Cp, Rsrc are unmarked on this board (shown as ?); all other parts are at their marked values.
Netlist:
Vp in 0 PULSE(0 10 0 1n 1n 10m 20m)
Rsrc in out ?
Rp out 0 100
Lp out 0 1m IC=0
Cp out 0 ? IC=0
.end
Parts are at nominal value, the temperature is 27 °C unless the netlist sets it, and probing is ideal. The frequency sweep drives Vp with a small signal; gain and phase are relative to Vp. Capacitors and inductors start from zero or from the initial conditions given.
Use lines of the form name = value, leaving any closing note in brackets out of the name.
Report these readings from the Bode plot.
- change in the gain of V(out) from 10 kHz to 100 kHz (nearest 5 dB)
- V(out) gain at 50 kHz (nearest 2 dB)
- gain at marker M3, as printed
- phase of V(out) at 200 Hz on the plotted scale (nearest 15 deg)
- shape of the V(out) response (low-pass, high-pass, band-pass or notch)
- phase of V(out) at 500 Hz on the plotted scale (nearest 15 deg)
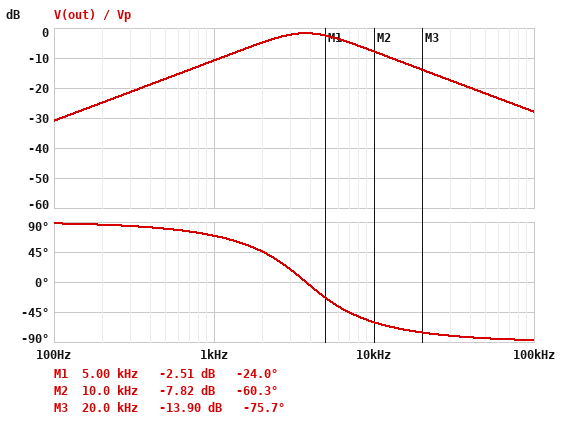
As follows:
change in the gain of V(out) from 10 kHz to 100 kHz = -20 dB
V(out) gain at 50 kHz = -22 dB
gain at marker M3, as printed = -13.90 dB
phase of V(out) at 200 Hz on the plotted scale = 90 deg
shape of the V(out) response = band-pass
phase of V(out) at 500 Hz on the plotted scale = 75 deg
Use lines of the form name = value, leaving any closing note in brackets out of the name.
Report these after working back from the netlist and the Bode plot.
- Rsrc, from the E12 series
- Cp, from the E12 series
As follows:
Rsrc, from the E12 series = 22 Ω
Cp, from the E12 series = 1.8 µF
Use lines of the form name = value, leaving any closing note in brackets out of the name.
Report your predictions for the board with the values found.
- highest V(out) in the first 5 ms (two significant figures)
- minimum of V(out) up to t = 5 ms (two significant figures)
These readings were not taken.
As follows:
highest V(out) in the first 5 ms = 5.1 V
minimum of V(out) up to t = 5 ms = -340 mV
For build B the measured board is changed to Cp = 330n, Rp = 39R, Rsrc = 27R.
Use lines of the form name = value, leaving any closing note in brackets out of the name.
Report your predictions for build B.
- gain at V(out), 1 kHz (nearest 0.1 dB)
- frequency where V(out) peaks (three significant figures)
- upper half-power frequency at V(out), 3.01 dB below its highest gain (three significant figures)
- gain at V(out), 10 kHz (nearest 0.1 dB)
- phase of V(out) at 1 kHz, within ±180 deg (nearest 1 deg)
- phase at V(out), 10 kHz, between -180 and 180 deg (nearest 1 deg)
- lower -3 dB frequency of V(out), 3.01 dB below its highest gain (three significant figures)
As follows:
gain at V(out), 1 kHz = -13.2 dB
frequency where V(out) peaks = 8.76 kHz
upper half-power frequency at V(out), 3.01 dB below its highest gain = 32.6 kHz
gain at V(out), 10 kHz = -4.6 dB
phase of V(out) at 1 kHz, within ±180 deg = 68 deg
phase at V(out), 10 kHz, between -180 and 180 deg = -4 deg
lower -3 dB frequency of V(out), 3.01 dB below its highest gain = 2.36 kHz
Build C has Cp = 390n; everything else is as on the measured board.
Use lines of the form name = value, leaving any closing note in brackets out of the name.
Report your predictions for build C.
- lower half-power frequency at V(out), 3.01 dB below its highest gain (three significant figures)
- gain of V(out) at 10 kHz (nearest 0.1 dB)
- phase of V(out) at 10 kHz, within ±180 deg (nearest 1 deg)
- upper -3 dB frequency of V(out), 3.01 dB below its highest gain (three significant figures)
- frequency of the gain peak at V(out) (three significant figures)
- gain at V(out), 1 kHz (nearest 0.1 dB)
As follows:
lower half-power frequency at V(out), 3.01 dB below its highest gain = 2.58 kHz
gain of V(out) at 10 kHz = -1.8 dB
phase of V(out) at 10 kHz, within ±180 deg = -9 deg
upper -3 dB frequency of V(out), 3.01 dB below its highest gain = 25.2 kHz
frequency of the gain peak at V(out) = 8.06 kHz
gain at V(out), 1 kHz = -11.3 dB
